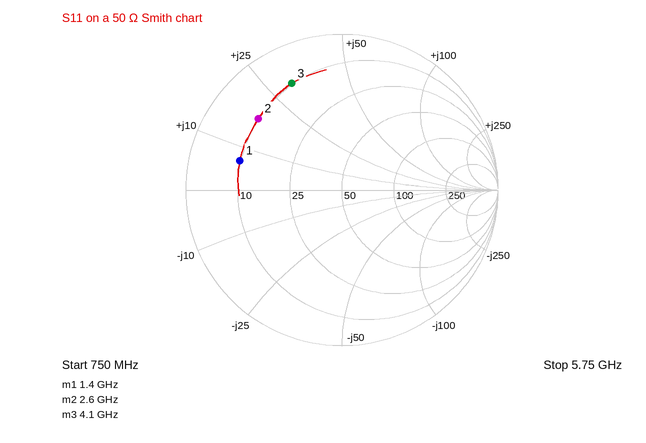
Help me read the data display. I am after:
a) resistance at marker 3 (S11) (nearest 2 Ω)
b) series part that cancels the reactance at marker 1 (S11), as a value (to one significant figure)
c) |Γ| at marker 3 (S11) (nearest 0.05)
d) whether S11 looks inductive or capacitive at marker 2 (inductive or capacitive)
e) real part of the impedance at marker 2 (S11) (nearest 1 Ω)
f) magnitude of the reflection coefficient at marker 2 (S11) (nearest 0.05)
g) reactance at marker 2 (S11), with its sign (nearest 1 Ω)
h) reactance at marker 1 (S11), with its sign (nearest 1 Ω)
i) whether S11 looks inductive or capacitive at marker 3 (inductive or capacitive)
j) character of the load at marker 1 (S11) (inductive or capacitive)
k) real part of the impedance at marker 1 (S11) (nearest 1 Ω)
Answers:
10 Ω
20 pF
0.75
inductive
10 Ω
0.70
+18 Ω
+7 Ω
inductive
inductive
10 Ω
